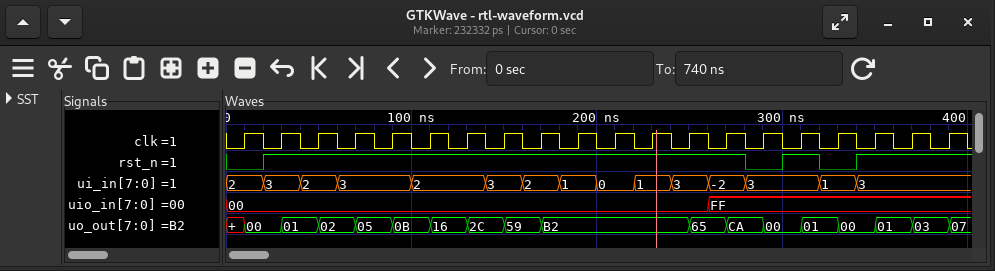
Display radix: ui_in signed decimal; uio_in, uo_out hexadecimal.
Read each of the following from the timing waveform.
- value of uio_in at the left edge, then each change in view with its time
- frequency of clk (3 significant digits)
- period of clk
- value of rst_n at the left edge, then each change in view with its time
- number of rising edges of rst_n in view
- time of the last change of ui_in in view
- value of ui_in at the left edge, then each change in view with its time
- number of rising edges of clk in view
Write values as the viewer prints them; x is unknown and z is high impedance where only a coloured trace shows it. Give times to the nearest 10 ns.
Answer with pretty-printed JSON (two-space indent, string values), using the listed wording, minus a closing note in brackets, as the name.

{
  "value of uio_in at the left edge, then each change in view with its time": "00, FF at 260 ns",
  "frequency of clk": "50.0 MHz",
  "period of clk": "20 ns",
  "value of rst_n at the left edge, then each change in view with its time": "0, 1 at 20 ns, 0 at 280 ns, 1 at 300 ns, 0 at 320 ns, 1 at 340 ns",
  "number of rising edges of rst_n in view": "3",
  "time of the last change of ui_in in view": "340 ns",
  "value of ui_in at the left edge, then each change in view with its time": "2, 3 at 20 ns, 2 at 40 ns, 3 at 60 ns, 2 at 100 ns, 3 at 140 ns, 2 at 160 ns, 1 at 180 ns, 0 at 200 ns, 1 at 220 ns, 3 at 240 ns, -2 at 260 ns, 3 at 280 ns, 1 at 320 ns, 3 at 340 ns",
  "number of rising edges of clk in view": "20"
}
